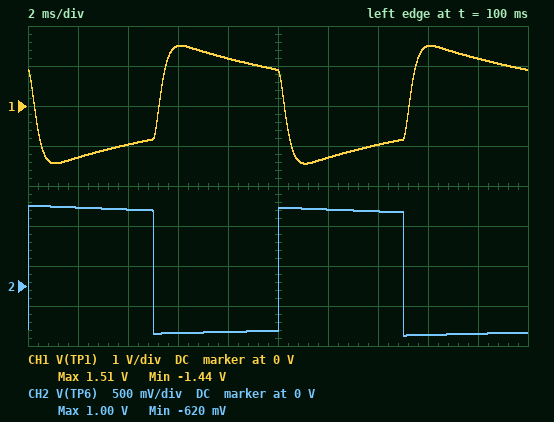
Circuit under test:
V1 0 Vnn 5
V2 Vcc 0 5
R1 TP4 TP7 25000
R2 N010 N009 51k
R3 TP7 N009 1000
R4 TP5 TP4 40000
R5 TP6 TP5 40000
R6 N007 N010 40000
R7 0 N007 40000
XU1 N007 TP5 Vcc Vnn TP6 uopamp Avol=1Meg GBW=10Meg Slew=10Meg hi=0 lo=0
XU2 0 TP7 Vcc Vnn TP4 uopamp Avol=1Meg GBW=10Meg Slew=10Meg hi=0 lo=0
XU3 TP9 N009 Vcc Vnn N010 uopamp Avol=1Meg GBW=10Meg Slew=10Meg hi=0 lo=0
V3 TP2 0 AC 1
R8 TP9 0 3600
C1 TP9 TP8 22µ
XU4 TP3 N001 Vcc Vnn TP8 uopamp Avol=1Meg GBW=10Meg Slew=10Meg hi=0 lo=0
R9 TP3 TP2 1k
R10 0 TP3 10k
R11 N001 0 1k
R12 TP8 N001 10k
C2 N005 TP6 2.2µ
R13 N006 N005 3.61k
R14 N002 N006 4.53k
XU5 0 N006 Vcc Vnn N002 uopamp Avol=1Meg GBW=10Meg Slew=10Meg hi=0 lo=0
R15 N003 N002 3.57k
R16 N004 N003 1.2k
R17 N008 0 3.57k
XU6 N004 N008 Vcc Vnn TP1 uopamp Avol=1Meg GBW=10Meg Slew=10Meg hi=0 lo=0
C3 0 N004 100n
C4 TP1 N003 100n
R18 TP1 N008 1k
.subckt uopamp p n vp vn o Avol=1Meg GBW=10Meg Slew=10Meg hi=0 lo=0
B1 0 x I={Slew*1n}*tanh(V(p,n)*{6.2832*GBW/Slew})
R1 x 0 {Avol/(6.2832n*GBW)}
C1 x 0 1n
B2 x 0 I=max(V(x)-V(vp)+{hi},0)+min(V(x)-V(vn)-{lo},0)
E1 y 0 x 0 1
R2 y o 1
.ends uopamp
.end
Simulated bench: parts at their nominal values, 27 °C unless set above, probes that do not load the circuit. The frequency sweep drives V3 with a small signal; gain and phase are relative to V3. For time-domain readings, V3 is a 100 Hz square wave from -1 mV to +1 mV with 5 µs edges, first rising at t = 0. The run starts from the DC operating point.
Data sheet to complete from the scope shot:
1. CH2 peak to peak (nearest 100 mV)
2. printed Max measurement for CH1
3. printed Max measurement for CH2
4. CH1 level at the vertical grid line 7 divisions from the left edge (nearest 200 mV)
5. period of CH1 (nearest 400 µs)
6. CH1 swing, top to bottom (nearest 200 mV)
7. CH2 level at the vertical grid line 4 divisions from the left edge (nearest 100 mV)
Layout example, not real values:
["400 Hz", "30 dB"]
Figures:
["1.6 V", "1.51 V", "1.00 V", "-1.0 V", "10.0 ms", "3.0 V", "-600 mV"]
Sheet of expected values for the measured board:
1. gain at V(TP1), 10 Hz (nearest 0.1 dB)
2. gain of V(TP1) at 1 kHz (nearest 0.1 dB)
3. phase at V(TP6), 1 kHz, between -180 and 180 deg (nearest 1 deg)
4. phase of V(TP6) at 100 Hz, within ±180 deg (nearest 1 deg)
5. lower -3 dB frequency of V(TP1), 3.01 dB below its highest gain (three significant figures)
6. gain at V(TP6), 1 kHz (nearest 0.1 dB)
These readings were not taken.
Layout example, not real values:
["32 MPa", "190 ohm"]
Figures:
["54.7 dB", "54.0 dB", "0 deg", "1 deg", "19.1 Hz", "57.7 dB"]
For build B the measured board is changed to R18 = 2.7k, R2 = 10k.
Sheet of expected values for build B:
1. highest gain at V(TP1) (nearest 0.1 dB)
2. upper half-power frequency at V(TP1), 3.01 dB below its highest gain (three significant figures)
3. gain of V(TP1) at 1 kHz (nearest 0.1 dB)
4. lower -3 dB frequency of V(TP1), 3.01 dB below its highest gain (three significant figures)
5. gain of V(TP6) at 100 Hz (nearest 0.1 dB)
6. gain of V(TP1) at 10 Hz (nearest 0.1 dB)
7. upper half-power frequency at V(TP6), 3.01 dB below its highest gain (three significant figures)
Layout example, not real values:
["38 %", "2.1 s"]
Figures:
["59.2 dB", "899 Hz", "54.6 dB", "28.4 Hz", "51.1 dB", "50.8 dB", "256 kHz"]
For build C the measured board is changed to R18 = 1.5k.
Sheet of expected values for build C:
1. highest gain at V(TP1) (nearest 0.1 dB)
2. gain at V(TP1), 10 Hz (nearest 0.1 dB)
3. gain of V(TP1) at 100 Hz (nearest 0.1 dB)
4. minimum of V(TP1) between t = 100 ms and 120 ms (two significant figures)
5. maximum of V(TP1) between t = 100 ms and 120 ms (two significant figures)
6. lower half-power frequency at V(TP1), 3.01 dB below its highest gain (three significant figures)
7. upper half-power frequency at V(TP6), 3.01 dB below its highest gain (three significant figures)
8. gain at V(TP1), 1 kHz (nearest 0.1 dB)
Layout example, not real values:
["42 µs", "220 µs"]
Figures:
["62.6 dB", "55.6 dB", "62.5 dB", "-1.7 V", "1.8 V", "19.5 Hz", "127 kHz", "56.0 dB"]
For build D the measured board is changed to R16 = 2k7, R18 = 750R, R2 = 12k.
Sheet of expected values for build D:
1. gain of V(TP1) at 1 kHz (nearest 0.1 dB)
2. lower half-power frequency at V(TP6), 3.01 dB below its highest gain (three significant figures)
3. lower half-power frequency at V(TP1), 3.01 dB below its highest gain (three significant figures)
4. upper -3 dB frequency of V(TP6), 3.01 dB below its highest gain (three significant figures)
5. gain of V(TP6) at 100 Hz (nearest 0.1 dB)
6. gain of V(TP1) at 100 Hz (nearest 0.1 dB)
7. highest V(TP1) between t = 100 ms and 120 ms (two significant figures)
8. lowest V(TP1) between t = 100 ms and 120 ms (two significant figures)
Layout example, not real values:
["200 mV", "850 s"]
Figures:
["42.2 dB", "2.01 Hz", "18.7 Hz", "244 kHz", "51.6 dB", "54.9 dB", "680 mV", "-650 mV"]
